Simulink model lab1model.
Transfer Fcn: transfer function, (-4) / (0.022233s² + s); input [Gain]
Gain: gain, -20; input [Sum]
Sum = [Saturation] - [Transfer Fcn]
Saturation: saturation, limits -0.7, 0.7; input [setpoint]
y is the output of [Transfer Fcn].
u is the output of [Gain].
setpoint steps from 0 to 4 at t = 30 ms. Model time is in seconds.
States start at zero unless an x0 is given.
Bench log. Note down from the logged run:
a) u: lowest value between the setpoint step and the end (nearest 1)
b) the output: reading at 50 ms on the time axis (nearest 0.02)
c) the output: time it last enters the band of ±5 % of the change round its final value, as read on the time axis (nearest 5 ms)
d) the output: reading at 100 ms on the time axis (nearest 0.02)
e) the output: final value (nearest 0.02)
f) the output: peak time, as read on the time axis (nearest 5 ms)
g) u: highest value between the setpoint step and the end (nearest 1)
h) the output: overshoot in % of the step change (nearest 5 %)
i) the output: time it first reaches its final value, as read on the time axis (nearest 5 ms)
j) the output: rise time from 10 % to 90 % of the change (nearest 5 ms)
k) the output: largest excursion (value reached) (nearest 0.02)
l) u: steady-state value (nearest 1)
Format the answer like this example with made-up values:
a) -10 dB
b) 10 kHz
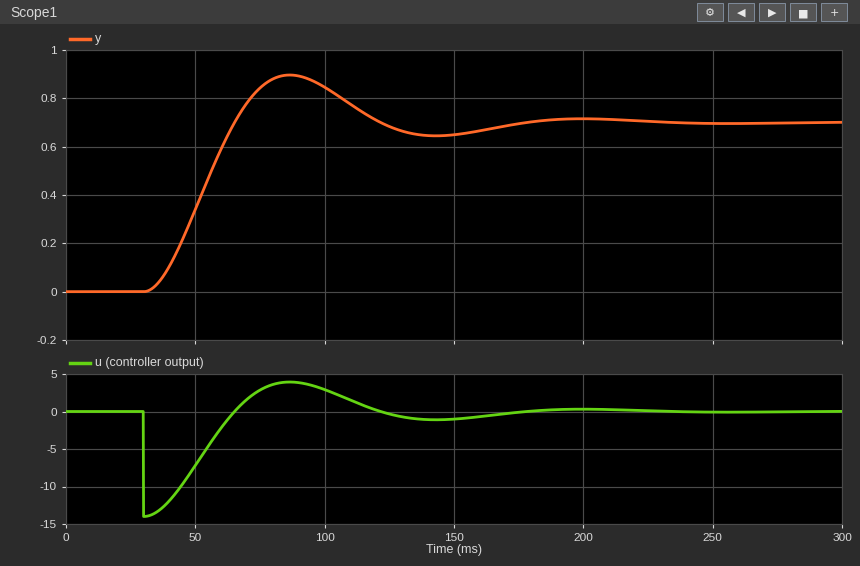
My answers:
a) -14
b) 0.34
c) 160 ms
d) 0.84
e) 0.70
f) 85 ms
g) 4
h) 30 %
i) 65 ms
j) 25 ms
k) 0.90
l) 0
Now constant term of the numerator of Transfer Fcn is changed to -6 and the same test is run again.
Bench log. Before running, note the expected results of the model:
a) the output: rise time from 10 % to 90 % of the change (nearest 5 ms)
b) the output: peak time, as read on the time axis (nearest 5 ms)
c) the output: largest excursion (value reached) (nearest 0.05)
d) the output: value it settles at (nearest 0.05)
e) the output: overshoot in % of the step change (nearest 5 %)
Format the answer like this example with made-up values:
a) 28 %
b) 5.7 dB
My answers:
a) 20 ms
b) 75 ms
c) 0.95
d) 0.70
e) 35 %
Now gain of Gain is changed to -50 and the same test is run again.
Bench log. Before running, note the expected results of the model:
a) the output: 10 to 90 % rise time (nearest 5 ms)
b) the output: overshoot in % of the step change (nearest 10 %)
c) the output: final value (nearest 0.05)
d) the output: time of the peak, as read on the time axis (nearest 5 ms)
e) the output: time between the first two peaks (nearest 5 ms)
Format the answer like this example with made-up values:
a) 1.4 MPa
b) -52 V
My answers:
a) 15 ms
b) 50 %
c) 0.70
d) 65 ms
e) 70 ms
